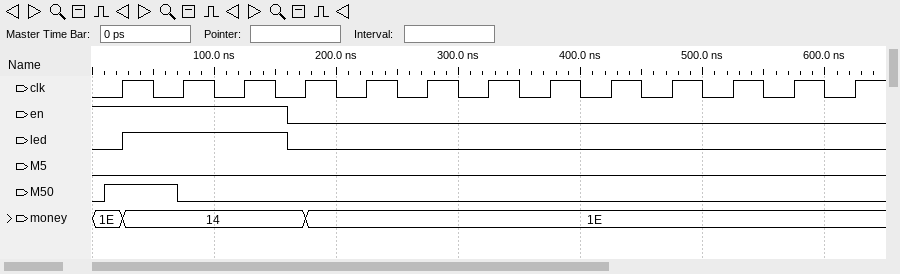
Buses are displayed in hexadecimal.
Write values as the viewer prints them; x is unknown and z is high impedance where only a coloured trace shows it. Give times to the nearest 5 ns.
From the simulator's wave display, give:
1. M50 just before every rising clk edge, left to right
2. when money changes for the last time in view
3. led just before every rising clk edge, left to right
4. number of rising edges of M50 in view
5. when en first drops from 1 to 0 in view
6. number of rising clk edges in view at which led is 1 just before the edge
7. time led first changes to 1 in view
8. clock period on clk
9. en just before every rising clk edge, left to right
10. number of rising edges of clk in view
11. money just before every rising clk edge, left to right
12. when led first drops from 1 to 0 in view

1 0 0 0 0 0 0 0 0 0 0 0 0
175 ns
0 1 1 0 0 0 0 0 0 0 0 0 0
1
160 ns
2
25 ns
50 ns
1 1 1 0 0 0 0 0 0 0 0 0 0
13
1E, 14, 14, 14, 1E, 1E, 1E, 1E, 1E, 1E, 1E, 1E, 1E
160 ns
